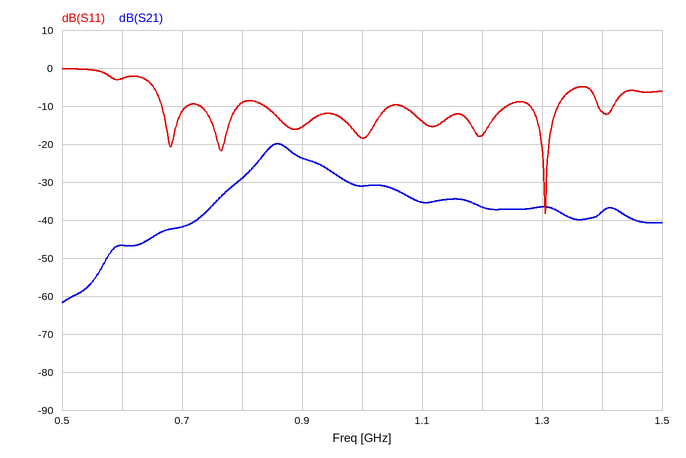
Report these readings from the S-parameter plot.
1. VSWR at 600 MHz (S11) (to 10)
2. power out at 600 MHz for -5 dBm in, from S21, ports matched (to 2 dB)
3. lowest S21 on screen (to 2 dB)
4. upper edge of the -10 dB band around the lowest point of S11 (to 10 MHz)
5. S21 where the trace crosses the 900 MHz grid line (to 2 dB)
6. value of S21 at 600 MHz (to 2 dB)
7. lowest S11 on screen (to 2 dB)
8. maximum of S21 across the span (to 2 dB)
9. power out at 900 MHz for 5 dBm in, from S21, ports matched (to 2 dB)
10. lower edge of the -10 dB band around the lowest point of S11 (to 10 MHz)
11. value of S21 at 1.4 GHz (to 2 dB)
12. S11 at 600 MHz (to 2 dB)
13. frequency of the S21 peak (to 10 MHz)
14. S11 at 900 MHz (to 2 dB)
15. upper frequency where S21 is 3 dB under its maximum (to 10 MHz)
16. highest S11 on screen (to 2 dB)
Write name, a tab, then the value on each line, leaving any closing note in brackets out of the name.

VSWR at 600 MHz (S11)	10
power out at 600 MHz for -5 dBm in, from S21, ports matched	-52 dBm
lowest S21 on screen	-62 dB
upper edge of the -10 dB band around the lowest point of S11	1.33 GHz
S21 where the trace crosses the 900 MHz grid line	-24 dB
value of S21 at 600 MHz	-46 dB
lowest S11 on screen	-38 dB
maximum of S21 across the span	-20 dB
power out at 900 MHz for 5 dBm in, from S21, ports matched	-18 dBm
lower edge of the -10 dB band around the lowest point of S11	1.28 GHz
value of S21 at 1.4 GHz	-38 dB
S11 at 600 MHz	-2 dB
frequency of the S21 peak	860 MHz
S11 at 900 MHz	-16 dB
upper frequency where S21 is 3 dB under its maximum	890 MHz
highest S11 on screen	0 dB
